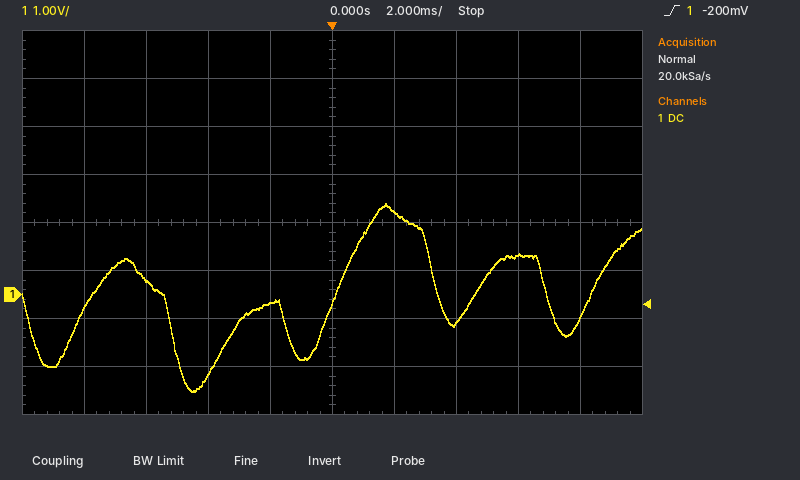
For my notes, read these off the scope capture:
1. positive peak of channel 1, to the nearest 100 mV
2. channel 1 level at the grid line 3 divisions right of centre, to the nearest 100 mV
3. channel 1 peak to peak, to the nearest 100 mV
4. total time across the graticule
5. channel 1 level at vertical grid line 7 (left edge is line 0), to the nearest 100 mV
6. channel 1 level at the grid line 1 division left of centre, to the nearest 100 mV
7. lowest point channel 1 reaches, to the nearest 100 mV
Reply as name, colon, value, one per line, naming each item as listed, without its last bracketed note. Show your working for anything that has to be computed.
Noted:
positive peak of channel 1, to the nearest 100 mV: 1.9 V
channel 1 level at the grid line 3 divisions right of centre, to the nearest 100 mV: 800 mV
channel 1 peak to peak, to the nearest 100 mV: 1.9 V − (-2.0 V) = 3.9 V
total time across the graticule: 20 ms
channel 1 level at vertical grid line 7 (left edge is line 0), to the nearest 100 mV: -600 mV
channel 1 level at the grid line 1 division left of centre, to the nearest 100 mV: -200 mV
lowest point channel 1 reaches, to the nearest 100 mV: -2.0 V
